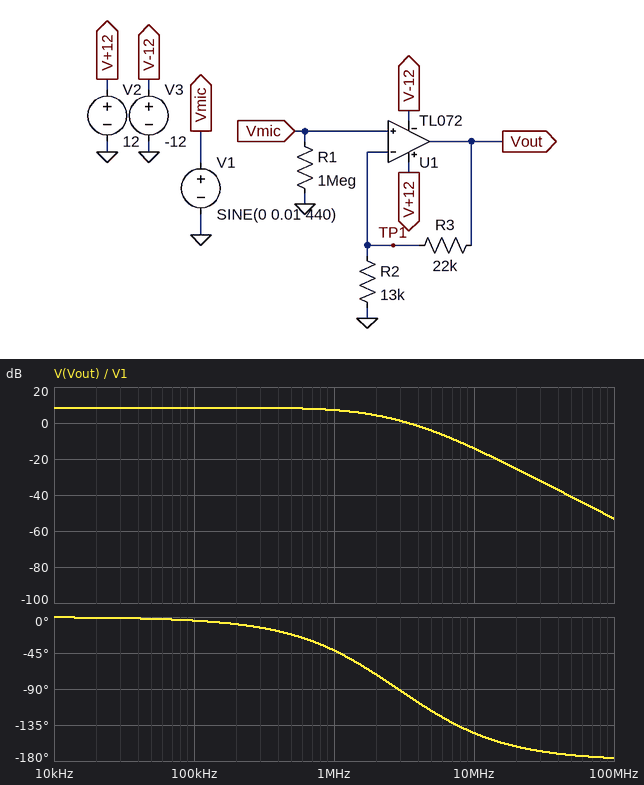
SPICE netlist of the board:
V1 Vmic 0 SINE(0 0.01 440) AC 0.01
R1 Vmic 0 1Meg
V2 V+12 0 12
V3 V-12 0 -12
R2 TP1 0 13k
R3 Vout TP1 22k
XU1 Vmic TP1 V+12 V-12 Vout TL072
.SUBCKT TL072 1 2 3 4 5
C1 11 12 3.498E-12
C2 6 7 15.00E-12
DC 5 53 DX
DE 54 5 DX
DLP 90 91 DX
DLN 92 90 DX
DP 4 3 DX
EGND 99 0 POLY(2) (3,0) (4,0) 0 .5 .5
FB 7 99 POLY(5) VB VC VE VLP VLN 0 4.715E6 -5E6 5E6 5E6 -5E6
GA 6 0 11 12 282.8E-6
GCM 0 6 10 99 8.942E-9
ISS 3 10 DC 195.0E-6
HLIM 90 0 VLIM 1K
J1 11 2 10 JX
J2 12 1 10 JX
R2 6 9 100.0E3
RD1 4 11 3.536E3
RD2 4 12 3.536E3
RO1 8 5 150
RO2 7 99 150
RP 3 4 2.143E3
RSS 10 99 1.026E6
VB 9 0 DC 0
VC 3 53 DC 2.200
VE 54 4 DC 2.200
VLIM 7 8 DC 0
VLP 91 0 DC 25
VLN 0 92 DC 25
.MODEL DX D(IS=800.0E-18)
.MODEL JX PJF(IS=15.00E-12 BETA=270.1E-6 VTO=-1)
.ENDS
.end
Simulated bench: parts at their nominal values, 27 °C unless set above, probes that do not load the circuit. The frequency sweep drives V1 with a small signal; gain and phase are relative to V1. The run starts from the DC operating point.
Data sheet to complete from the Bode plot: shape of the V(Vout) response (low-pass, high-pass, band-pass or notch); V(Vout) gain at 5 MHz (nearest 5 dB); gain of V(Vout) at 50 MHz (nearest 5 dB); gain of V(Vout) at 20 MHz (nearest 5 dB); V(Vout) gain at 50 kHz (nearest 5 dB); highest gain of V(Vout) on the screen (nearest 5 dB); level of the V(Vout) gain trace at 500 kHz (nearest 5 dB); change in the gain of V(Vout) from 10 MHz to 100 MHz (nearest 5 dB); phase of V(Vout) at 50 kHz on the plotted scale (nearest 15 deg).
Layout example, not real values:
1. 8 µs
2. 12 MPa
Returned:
1. low-pass
2. -5 dB
3. -40 dB
4. -25 dB
5. 10 dB
6. 10 dB
7. 10 dB
8. -40 dB
9. 0 deg
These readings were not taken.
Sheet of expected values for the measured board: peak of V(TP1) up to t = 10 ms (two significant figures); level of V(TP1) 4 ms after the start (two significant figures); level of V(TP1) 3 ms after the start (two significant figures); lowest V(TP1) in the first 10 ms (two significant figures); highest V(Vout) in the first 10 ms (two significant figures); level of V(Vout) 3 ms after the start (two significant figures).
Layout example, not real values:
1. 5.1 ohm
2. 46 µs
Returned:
1. 10 mV
2. -10 mV
3. 9.1 mV
4. -10 mV
5. 27 mV
6. 24 mV
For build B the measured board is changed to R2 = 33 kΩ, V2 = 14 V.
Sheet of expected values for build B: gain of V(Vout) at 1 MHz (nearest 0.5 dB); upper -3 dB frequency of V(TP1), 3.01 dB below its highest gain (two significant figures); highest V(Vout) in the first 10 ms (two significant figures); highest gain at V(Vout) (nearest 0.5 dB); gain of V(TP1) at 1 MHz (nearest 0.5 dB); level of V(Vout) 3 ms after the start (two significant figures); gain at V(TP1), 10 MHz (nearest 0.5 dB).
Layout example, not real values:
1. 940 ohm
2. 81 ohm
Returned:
1. 4.0 dB
2. 2.8 MHz
3. 17 mV
4. 4.5 dB
5. -0.5 dB
6. 15 mV
7. -18.0 dB
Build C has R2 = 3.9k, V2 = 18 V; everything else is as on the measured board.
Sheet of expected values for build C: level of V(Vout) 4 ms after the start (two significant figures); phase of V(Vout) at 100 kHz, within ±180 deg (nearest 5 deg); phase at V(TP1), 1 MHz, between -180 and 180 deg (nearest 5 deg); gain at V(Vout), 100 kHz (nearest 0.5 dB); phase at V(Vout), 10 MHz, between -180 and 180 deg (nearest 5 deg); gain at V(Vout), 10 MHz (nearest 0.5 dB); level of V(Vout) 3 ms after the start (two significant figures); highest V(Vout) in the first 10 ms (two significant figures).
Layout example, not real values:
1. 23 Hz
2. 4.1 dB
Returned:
1. -66 mV
2. -10 deg
3. -70 deg
4. 16.5 dB
5. -145 deg
6. -14.5 dB
7. 61 mV
8. 67 mV
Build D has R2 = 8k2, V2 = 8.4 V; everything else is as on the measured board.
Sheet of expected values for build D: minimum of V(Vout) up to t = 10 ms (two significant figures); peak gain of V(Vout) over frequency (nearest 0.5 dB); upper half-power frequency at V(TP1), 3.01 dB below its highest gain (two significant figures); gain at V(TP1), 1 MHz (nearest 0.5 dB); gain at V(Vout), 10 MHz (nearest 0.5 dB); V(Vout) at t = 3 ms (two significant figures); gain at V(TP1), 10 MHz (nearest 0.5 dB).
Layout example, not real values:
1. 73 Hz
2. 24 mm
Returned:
1. -37 mV
2. 11.5 dB
3. 1.1 MHz
4. -2.5 dB
5. -14.5 dB
6. 33 mV
7. -25.5 dB
